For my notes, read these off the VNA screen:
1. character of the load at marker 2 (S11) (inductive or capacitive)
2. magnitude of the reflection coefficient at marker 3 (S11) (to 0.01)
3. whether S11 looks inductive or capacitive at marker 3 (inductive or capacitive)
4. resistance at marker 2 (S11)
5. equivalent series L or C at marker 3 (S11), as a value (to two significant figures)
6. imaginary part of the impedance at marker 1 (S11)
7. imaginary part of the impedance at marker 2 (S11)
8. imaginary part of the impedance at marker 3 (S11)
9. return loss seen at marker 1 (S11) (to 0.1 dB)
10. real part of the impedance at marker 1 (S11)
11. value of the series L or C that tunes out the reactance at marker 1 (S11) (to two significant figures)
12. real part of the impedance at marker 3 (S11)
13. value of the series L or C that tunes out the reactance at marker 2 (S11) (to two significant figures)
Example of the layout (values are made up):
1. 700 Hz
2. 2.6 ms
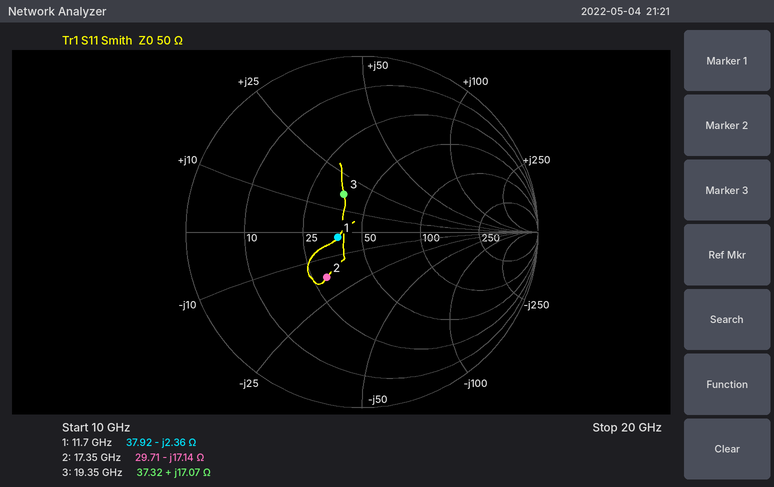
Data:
1. capacitive
2. 0.24
3. inductive
4. 29.71 Ω
5. 140 pH
6. -2.36 Ω
7. -17.14 Ω
8. +17.07 Ω
9. 17.1 dB
10. 37.92 Ω
11. 32 pH
12. 37.32 Ω
13. 160 pH
